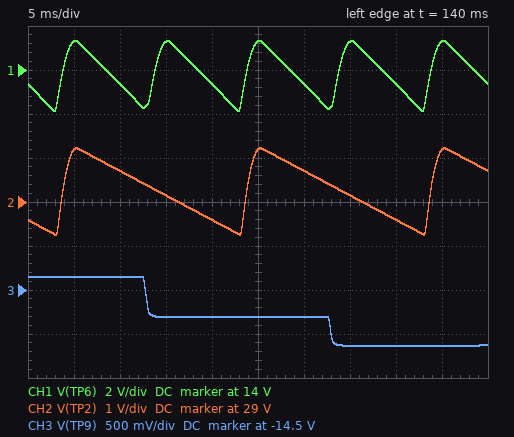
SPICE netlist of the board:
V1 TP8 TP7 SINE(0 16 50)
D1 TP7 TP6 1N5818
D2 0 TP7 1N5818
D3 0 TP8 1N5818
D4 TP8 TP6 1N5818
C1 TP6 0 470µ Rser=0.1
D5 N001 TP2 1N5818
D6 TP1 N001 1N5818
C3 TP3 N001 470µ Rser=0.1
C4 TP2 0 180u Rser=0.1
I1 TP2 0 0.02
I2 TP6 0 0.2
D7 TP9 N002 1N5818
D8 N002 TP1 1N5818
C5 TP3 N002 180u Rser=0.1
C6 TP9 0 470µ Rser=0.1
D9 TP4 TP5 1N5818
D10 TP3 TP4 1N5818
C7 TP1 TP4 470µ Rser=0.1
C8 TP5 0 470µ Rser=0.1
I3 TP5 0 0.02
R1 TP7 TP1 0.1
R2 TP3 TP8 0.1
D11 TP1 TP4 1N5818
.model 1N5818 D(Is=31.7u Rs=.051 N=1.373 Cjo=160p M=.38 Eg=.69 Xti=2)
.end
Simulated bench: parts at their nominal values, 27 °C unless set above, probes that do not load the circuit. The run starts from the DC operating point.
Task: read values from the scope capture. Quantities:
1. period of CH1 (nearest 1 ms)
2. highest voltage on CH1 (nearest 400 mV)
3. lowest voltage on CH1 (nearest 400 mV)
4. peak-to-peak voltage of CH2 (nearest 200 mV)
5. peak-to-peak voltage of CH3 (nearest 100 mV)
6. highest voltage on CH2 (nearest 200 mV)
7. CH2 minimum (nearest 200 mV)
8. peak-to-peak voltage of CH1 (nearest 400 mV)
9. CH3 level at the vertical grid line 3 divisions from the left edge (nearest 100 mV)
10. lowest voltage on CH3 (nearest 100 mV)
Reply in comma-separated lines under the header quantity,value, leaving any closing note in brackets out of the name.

quantity,value
period of CH1,10 ms
highest voltage on CH1,15.2 V
lowest voltage on CH1,12.0 V
peak-to-peak voltage of CH2,2.0 V
peak-to-peak voltage of CH3,800 mV
highest voltage on CH2,30.2 V
CH2 minimum,28.2 V
peak-to-peak voltage of CH1,3.2 V
CH3 level at the vertical grid line 3 divisions from the left edge,-14.8 V
lowest voltage on CH3,-15.1 V
